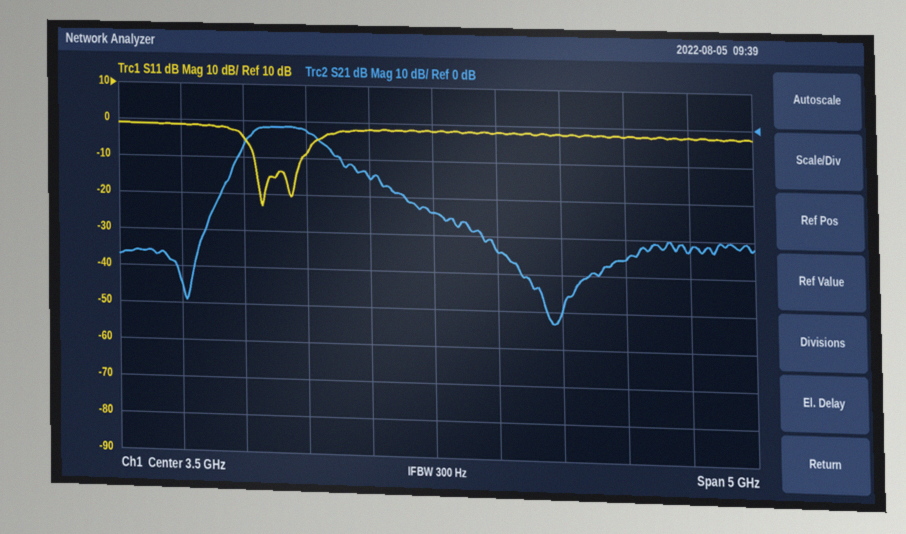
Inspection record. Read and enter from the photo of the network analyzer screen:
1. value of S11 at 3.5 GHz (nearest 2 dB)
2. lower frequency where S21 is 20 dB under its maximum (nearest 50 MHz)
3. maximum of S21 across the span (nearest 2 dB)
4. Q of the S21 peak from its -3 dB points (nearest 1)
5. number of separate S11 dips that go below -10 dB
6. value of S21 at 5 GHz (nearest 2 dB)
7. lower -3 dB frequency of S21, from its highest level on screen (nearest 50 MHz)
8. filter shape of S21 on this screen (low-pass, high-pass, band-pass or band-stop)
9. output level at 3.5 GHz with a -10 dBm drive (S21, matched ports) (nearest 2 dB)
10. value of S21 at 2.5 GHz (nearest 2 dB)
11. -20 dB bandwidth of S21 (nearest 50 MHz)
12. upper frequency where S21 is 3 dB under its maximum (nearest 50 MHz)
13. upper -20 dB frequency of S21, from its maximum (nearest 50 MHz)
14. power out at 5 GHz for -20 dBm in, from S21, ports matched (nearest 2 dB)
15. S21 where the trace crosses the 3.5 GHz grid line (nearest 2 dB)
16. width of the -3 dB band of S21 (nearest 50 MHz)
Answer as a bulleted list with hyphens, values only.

- -2 dB
- 1.80 GHz
- -2 dB
- 4
- 2
- -36 dB
- 2.05 GHz
- band-pass
- -34 dBm
- -2 dB
- 1.55 GHz
- 2.60 GHz
- 3.35 GHz
- -56 dBm
- -24 dB
- 550 MHz
